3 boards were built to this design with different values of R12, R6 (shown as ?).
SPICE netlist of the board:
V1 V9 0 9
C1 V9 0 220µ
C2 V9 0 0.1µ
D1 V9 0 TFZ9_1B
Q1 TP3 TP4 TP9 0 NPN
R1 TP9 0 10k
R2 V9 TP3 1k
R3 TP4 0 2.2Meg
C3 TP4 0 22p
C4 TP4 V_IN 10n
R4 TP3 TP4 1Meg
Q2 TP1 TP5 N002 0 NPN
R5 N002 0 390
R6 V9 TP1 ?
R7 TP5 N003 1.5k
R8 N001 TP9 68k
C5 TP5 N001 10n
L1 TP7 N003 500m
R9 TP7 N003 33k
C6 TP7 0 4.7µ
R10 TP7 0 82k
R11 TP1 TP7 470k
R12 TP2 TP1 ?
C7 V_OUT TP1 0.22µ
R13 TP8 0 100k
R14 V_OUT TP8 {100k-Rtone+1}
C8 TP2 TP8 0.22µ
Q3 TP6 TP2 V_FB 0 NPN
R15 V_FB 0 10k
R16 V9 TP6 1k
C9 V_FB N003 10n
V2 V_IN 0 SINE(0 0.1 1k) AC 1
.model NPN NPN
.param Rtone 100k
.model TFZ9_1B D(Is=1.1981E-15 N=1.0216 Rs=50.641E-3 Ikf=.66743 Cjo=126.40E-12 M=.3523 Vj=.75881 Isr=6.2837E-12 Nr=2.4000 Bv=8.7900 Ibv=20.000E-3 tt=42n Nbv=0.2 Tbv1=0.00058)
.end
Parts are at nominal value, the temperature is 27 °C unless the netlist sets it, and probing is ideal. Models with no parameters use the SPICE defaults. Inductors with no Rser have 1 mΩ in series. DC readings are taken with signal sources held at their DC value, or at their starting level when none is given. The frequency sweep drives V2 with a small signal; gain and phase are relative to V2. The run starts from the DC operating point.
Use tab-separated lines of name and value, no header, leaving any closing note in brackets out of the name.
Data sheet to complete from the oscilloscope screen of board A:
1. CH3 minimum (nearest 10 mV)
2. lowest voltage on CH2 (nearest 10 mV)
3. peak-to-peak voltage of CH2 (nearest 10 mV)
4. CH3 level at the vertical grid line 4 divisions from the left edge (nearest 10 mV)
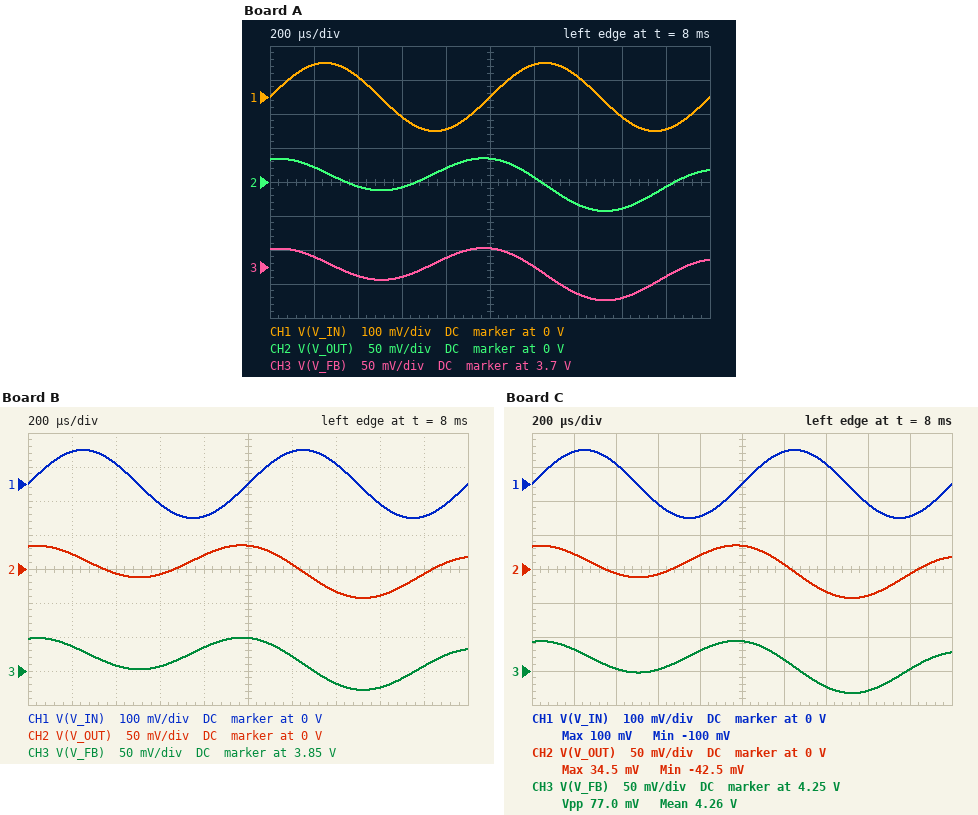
CH3 minimum	3.65 V
lowest voltage on CH2	-40 mV
peak-to-peak voltage of CH2	80 mV
CH3 level at the vertical grid line 4 divisions from the left edge	3.71 V
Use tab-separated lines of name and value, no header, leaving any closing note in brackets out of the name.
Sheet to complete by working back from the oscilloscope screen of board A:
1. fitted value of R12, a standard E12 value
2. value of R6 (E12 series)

fitted value of R12, a standard E12 value	330 kΩ
value of R6	27 kΩ
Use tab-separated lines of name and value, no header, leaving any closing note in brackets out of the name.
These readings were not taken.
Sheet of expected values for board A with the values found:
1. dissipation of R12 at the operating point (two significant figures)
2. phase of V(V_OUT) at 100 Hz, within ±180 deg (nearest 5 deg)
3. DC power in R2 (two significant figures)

dissipation of R12 at the operating point	4.4 µW
phase of V(V_OUT) at 100 Hz, within ±180 deg	-90 deg
DC power in R2	98 µW
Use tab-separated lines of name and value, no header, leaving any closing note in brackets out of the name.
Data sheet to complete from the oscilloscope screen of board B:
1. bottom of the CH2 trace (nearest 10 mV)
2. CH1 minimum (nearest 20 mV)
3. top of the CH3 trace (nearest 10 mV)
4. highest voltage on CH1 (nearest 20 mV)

bottom of the CH2 trace	-40 mV
CH1 minimum	-100 mV
top of the CH3 trace	3.90 V
highest voltage on CH1	100 mV
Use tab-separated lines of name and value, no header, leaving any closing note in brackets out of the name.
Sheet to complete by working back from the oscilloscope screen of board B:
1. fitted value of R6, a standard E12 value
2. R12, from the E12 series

fitted value of R6, a standard E12 value	27 kΩ
R12, from the E12 series	270 kΩ
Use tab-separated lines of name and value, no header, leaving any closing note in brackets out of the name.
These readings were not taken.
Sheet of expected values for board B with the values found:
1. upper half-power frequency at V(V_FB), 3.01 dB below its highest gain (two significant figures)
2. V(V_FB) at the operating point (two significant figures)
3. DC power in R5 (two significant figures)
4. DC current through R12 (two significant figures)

upper half-power frequency at V(V_FB), 3.01 dB below its highest gain	430 Hz
V(V_FB) at the operating point	3.9 V
DC power in R5	4.8 µW
DC current through R12	3.8 µA
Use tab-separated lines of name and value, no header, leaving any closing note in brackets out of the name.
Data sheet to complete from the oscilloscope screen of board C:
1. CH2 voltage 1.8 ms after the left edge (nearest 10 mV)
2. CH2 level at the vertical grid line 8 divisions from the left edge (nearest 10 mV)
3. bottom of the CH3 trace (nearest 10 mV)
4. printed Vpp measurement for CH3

CH2 voltage 1.8 ms after the left edge	-10 mV
CH2 level at the vertical grid line 8 divisions from the left edge	-40 mV
bottom of the CH3 trace	4.22 V
printed Vpp measurement for CH3	77.0 mV
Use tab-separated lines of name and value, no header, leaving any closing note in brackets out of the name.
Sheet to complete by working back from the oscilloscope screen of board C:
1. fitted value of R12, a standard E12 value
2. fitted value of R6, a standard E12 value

fitted value of R12, a standard E12 value	150 kΩ
fitted value of R6, a standard E12 value	27 kΩ
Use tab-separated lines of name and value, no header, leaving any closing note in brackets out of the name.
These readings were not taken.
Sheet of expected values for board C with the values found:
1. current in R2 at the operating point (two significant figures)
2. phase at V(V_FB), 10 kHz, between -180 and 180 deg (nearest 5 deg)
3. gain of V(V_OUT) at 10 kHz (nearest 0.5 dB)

current in R2 at the operating point	310 µA
phase at V(V_FB), 10 kHz, between -180 and 180 deg	130 deg
gain of V(V_OUT) at 10 kHz	-30.0 dB
